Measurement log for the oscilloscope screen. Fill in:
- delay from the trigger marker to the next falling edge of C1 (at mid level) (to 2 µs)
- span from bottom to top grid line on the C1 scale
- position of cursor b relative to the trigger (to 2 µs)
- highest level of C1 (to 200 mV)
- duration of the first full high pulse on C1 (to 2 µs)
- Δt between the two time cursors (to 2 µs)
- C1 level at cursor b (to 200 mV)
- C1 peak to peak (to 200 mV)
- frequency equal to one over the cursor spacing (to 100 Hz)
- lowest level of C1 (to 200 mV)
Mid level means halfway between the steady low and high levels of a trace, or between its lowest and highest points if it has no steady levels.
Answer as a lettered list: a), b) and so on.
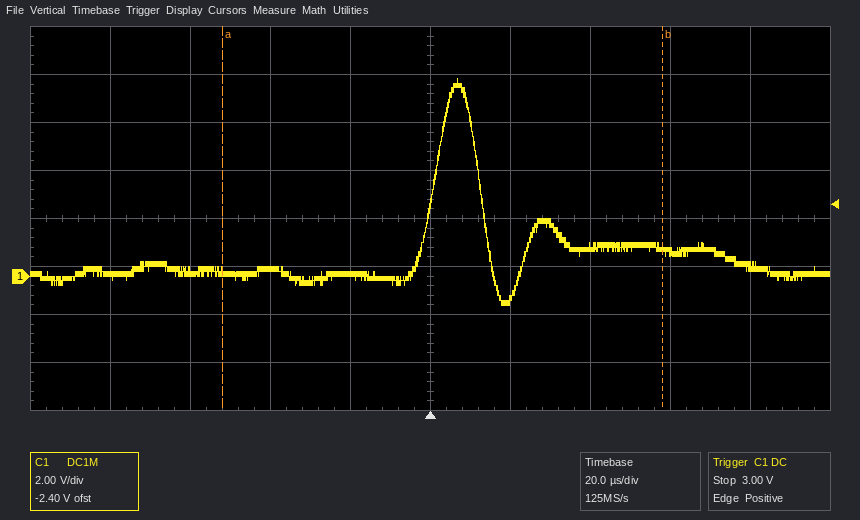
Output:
a) 12 µs
b) 16 V
c) +58 µs
d) 8.2 V
e) 12 µs
f) 110 µs
g) 1.0 V
h) 9.4 V
i) 9.1 kHz
j) -1.2 V
